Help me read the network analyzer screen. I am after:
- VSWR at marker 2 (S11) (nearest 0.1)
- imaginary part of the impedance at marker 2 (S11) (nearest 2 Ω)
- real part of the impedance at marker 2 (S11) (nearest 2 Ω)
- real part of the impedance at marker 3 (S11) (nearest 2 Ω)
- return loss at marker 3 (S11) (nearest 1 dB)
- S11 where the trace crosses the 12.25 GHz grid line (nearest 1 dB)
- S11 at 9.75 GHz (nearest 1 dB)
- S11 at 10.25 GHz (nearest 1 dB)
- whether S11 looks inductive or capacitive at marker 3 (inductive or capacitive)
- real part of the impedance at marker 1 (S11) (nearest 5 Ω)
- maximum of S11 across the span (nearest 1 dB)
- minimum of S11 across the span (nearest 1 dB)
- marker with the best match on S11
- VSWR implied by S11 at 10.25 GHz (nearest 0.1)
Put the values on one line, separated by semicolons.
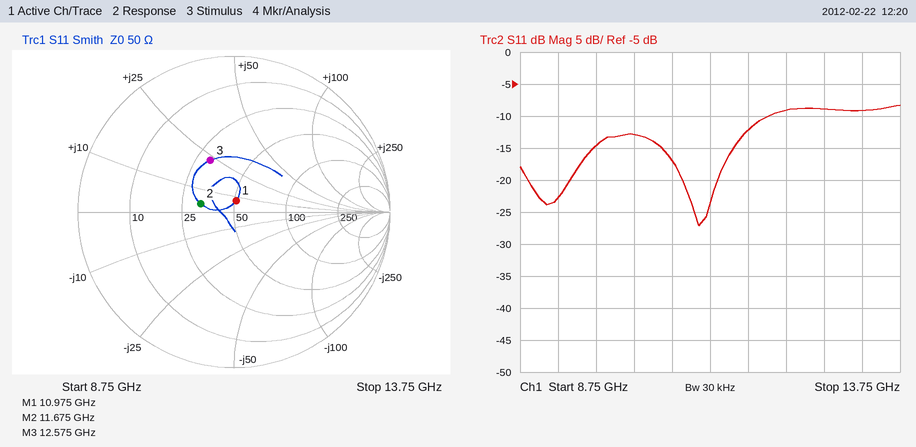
1.6; +4 Ω; 32 Ω; 30 Ω; 9 dB; -9 dB; -15 dB; -13 dB; inductive; 50 Ω; -8 dB; -27 dB; marker 1; 1.6
